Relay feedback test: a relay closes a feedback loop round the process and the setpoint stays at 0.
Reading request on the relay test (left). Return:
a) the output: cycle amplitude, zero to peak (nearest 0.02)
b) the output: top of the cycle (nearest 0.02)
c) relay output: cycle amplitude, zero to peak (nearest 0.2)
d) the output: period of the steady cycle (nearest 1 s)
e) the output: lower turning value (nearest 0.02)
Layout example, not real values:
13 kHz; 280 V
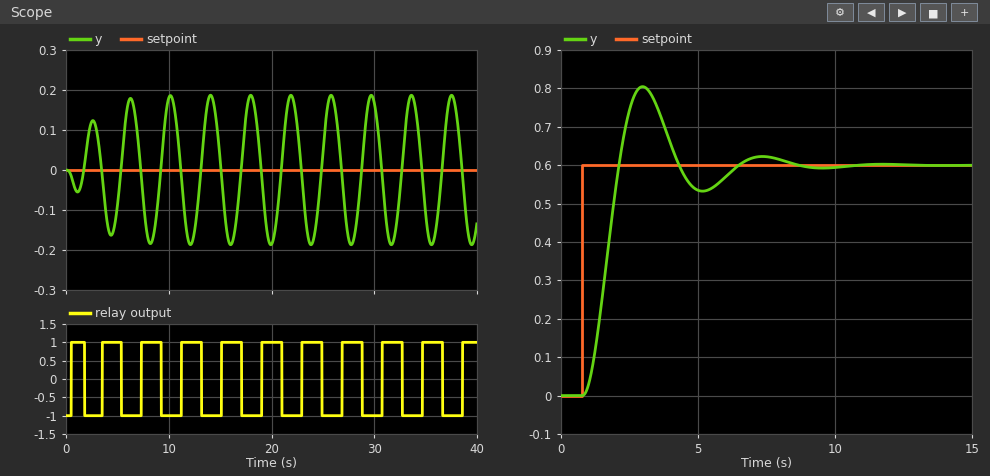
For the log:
0.18; 0.18; 1.0; 4 s; -0.18
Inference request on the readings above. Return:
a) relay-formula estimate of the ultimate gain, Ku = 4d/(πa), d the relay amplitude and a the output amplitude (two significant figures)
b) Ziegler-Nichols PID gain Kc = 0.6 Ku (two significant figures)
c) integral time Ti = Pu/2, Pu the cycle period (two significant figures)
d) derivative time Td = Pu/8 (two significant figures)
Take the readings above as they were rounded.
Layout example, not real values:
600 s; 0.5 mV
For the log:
7.1; 4.3; 2.0 s; 0.50 s
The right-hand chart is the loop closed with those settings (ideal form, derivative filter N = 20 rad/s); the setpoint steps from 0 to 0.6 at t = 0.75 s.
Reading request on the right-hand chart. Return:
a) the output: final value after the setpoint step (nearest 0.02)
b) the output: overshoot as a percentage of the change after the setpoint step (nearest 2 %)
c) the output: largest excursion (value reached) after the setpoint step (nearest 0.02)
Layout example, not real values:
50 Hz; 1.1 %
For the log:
0.60; 34 %; 0.80
